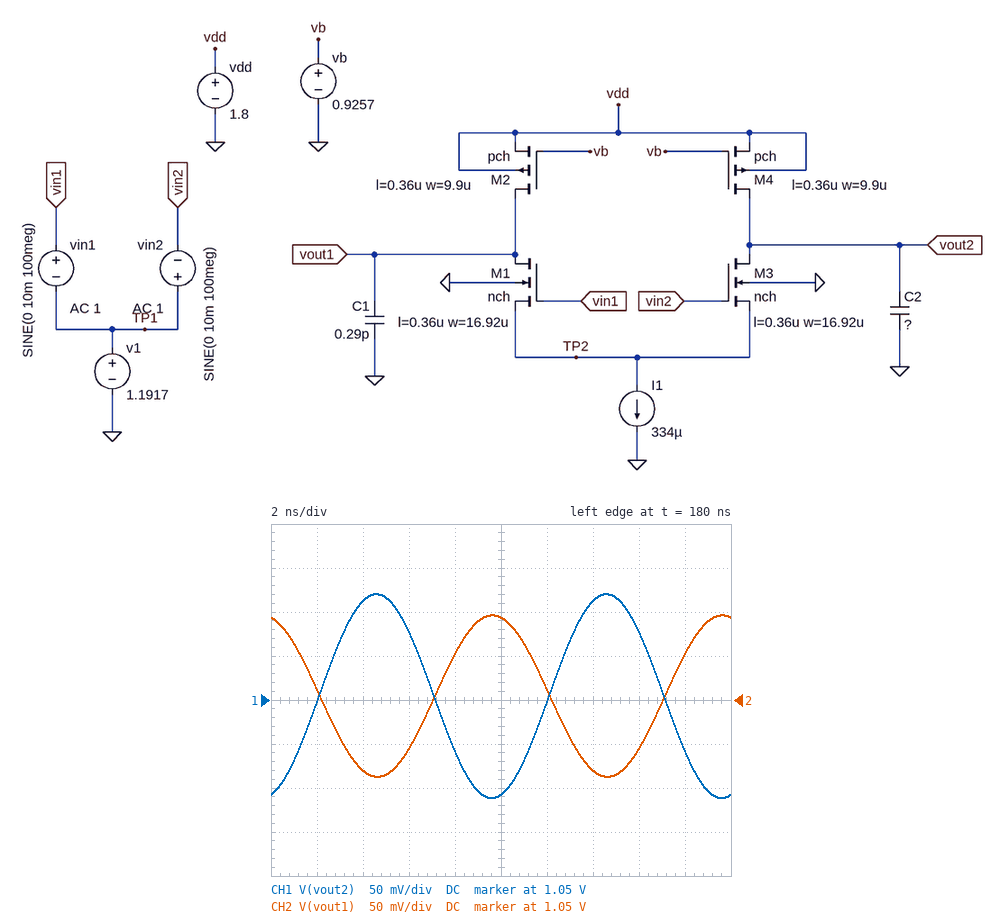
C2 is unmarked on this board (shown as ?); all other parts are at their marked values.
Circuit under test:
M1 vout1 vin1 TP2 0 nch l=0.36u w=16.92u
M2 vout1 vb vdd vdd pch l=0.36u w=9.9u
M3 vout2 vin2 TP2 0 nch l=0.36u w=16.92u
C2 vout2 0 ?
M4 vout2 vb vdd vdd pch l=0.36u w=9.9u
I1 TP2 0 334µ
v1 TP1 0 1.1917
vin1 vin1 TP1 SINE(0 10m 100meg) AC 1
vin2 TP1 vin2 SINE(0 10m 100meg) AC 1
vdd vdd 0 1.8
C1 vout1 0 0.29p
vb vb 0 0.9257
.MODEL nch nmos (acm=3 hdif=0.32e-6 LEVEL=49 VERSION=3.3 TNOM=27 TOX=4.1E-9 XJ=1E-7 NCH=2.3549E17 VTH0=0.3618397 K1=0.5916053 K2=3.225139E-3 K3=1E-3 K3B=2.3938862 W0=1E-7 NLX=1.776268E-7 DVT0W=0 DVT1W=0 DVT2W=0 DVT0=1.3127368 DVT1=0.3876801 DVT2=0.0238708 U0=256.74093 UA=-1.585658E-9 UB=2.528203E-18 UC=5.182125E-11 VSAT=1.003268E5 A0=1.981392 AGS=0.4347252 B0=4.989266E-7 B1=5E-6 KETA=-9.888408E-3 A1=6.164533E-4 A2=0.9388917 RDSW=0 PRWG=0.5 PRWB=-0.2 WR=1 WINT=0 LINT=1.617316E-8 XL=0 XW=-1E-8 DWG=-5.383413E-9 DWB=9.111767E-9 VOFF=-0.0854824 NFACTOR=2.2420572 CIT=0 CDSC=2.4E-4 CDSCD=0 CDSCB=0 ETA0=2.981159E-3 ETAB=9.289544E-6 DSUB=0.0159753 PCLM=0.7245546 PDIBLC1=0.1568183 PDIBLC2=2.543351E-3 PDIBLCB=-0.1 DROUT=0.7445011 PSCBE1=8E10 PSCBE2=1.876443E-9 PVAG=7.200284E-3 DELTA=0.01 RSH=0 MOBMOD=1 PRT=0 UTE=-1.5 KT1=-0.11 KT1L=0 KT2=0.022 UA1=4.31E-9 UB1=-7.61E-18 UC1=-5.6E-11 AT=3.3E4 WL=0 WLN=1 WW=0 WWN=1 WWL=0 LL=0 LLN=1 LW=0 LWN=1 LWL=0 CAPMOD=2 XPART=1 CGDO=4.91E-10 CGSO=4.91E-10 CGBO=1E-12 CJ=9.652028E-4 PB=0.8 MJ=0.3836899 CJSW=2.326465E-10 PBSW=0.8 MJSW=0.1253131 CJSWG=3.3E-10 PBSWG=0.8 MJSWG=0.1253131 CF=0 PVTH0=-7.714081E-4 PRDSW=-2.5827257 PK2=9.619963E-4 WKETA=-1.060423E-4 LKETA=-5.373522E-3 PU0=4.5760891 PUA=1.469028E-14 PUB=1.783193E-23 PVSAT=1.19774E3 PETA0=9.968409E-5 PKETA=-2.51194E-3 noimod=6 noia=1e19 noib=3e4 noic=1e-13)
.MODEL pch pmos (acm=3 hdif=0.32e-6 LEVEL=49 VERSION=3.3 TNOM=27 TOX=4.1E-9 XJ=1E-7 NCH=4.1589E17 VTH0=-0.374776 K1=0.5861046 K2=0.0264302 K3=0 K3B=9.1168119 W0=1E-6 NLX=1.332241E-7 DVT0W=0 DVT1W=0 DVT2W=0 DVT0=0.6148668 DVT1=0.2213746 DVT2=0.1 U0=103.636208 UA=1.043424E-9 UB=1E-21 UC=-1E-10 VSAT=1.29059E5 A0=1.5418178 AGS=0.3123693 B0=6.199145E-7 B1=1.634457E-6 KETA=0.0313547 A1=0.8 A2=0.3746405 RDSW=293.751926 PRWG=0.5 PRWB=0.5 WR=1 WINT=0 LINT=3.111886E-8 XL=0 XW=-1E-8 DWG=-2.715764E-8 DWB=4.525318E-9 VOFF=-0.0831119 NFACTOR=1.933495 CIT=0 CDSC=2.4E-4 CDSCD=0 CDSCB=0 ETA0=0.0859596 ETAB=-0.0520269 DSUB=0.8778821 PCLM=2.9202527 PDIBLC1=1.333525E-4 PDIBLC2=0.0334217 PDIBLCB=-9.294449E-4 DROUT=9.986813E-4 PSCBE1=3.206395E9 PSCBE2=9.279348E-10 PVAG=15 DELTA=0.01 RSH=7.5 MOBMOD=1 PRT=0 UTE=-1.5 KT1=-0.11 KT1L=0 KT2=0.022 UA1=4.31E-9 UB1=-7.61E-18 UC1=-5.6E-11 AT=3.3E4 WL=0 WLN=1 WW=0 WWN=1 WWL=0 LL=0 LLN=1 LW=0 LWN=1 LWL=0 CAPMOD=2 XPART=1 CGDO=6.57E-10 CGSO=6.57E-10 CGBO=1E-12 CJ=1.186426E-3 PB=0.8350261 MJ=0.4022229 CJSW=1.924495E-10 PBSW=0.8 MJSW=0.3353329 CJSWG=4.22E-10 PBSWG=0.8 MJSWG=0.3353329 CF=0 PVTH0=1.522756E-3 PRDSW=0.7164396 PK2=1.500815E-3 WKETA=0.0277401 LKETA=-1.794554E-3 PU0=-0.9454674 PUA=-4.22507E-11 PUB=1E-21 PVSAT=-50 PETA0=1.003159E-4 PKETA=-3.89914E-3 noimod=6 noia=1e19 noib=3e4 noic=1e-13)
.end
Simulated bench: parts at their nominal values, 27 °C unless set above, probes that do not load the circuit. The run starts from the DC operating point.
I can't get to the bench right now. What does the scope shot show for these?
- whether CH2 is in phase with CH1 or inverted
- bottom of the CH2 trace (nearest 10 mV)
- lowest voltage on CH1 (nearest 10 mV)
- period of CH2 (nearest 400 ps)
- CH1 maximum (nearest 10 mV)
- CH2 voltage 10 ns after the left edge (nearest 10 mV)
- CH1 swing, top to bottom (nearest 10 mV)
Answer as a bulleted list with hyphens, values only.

- inverted
- 960 mV
- 940 mV
- 10.0 ns
- 1.17 V
- 1.14 V
- 230 mV
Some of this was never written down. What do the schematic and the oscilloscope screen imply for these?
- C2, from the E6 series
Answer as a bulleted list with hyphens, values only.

- 220 fF
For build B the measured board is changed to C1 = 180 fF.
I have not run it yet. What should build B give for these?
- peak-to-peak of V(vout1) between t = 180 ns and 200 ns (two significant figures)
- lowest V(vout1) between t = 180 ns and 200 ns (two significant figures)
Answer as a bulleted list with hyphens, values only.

- 270 mV
- 920 mV
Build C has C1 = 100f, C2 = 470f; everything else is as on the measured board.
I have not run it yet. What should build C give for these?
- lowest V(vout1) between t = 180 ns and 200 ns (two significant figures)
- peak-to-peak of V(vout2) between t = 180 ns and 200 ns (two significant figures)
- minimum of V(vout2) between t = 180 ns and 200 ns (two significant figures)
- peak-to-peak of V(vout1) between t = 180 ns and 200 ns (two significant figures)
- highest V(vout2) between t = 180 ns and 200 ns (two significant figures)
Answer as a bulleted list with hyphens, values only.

- 850 mV
- 120 mV
- 990 mV
- 410 mV
- 1.1 V
